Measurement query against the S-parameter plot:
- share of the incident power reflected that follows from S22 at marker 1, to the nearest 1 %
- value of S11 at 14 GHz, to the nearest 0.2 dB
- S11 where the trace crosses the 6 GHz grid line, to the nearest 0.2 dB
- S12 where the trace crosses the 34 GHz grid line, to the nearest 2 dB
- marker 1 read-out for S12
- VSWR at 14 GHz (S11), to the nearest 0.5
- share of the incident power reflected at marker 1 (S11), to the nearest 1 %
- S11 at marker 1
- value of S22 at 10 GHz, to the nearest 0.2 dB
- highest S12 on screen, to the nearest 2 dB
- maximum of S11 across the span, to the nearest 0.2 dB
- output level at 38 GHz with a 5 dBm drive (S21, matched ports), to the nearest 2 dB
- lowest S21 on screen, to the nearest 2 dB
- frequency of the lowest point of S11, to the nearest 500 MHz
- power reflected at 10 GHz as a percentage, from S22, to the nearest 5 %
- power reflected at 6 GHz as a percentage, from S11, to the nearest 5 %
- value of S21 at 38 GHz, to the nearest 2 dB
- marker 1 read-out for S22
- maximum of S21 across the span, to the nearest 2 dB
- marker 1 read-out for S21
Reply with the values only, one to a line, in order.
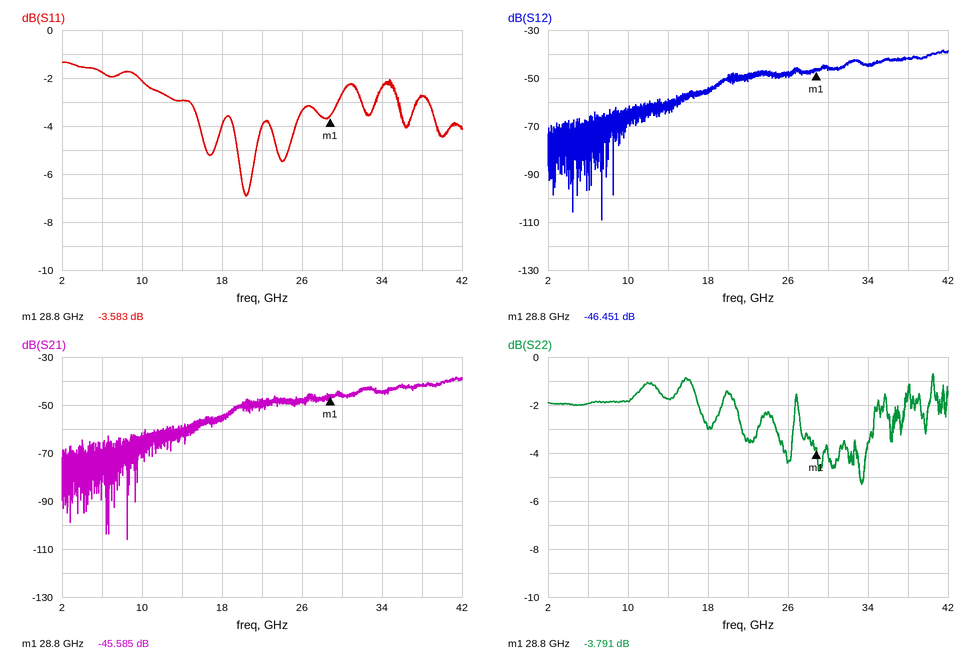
42 %
-3.0 dB
-1.8 dB
-44 dB
-46.451 dB
6.0
44 %
-3.583 dB
-1.8 dB
-38 dB
-1.4 dB
-36 dBm
-106 dB
20.5 GHz
65 %
65 %
-42 dB
-3.791 dB
-38 dB
-45.585 dB
